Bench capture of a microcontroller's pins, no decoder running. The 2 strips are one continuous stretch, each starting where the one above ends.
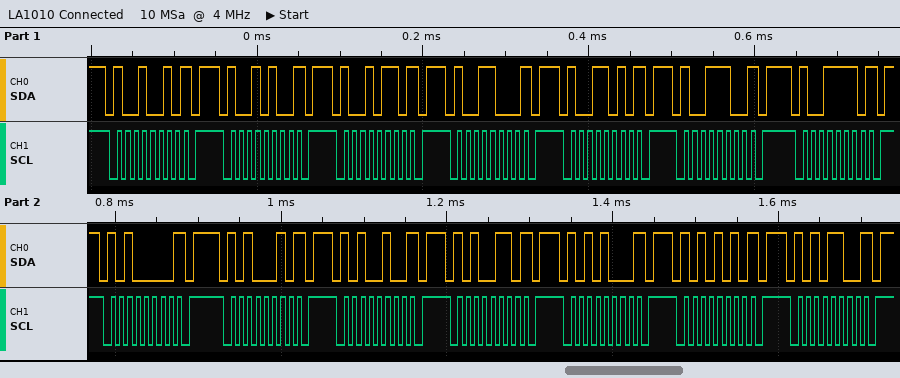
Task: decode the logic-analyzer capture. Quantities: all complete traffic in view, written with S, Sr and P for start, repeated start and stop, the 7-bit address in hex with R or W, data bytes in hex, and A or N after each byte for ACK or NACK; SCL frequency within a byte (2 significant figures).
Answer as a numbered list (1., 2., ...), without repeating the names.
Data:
1. S 49W N P S 4AW N P S 4BW N P S 4CW N P S 4DW N P S 4EW N P S 4FW N P S 50W N P S 51W N P S 52W N P S 53W N P S 54W N P S 55W N P S 56W N P
2. 100 kHz
